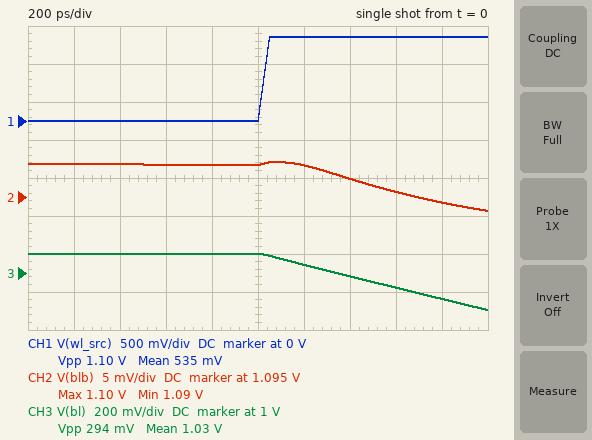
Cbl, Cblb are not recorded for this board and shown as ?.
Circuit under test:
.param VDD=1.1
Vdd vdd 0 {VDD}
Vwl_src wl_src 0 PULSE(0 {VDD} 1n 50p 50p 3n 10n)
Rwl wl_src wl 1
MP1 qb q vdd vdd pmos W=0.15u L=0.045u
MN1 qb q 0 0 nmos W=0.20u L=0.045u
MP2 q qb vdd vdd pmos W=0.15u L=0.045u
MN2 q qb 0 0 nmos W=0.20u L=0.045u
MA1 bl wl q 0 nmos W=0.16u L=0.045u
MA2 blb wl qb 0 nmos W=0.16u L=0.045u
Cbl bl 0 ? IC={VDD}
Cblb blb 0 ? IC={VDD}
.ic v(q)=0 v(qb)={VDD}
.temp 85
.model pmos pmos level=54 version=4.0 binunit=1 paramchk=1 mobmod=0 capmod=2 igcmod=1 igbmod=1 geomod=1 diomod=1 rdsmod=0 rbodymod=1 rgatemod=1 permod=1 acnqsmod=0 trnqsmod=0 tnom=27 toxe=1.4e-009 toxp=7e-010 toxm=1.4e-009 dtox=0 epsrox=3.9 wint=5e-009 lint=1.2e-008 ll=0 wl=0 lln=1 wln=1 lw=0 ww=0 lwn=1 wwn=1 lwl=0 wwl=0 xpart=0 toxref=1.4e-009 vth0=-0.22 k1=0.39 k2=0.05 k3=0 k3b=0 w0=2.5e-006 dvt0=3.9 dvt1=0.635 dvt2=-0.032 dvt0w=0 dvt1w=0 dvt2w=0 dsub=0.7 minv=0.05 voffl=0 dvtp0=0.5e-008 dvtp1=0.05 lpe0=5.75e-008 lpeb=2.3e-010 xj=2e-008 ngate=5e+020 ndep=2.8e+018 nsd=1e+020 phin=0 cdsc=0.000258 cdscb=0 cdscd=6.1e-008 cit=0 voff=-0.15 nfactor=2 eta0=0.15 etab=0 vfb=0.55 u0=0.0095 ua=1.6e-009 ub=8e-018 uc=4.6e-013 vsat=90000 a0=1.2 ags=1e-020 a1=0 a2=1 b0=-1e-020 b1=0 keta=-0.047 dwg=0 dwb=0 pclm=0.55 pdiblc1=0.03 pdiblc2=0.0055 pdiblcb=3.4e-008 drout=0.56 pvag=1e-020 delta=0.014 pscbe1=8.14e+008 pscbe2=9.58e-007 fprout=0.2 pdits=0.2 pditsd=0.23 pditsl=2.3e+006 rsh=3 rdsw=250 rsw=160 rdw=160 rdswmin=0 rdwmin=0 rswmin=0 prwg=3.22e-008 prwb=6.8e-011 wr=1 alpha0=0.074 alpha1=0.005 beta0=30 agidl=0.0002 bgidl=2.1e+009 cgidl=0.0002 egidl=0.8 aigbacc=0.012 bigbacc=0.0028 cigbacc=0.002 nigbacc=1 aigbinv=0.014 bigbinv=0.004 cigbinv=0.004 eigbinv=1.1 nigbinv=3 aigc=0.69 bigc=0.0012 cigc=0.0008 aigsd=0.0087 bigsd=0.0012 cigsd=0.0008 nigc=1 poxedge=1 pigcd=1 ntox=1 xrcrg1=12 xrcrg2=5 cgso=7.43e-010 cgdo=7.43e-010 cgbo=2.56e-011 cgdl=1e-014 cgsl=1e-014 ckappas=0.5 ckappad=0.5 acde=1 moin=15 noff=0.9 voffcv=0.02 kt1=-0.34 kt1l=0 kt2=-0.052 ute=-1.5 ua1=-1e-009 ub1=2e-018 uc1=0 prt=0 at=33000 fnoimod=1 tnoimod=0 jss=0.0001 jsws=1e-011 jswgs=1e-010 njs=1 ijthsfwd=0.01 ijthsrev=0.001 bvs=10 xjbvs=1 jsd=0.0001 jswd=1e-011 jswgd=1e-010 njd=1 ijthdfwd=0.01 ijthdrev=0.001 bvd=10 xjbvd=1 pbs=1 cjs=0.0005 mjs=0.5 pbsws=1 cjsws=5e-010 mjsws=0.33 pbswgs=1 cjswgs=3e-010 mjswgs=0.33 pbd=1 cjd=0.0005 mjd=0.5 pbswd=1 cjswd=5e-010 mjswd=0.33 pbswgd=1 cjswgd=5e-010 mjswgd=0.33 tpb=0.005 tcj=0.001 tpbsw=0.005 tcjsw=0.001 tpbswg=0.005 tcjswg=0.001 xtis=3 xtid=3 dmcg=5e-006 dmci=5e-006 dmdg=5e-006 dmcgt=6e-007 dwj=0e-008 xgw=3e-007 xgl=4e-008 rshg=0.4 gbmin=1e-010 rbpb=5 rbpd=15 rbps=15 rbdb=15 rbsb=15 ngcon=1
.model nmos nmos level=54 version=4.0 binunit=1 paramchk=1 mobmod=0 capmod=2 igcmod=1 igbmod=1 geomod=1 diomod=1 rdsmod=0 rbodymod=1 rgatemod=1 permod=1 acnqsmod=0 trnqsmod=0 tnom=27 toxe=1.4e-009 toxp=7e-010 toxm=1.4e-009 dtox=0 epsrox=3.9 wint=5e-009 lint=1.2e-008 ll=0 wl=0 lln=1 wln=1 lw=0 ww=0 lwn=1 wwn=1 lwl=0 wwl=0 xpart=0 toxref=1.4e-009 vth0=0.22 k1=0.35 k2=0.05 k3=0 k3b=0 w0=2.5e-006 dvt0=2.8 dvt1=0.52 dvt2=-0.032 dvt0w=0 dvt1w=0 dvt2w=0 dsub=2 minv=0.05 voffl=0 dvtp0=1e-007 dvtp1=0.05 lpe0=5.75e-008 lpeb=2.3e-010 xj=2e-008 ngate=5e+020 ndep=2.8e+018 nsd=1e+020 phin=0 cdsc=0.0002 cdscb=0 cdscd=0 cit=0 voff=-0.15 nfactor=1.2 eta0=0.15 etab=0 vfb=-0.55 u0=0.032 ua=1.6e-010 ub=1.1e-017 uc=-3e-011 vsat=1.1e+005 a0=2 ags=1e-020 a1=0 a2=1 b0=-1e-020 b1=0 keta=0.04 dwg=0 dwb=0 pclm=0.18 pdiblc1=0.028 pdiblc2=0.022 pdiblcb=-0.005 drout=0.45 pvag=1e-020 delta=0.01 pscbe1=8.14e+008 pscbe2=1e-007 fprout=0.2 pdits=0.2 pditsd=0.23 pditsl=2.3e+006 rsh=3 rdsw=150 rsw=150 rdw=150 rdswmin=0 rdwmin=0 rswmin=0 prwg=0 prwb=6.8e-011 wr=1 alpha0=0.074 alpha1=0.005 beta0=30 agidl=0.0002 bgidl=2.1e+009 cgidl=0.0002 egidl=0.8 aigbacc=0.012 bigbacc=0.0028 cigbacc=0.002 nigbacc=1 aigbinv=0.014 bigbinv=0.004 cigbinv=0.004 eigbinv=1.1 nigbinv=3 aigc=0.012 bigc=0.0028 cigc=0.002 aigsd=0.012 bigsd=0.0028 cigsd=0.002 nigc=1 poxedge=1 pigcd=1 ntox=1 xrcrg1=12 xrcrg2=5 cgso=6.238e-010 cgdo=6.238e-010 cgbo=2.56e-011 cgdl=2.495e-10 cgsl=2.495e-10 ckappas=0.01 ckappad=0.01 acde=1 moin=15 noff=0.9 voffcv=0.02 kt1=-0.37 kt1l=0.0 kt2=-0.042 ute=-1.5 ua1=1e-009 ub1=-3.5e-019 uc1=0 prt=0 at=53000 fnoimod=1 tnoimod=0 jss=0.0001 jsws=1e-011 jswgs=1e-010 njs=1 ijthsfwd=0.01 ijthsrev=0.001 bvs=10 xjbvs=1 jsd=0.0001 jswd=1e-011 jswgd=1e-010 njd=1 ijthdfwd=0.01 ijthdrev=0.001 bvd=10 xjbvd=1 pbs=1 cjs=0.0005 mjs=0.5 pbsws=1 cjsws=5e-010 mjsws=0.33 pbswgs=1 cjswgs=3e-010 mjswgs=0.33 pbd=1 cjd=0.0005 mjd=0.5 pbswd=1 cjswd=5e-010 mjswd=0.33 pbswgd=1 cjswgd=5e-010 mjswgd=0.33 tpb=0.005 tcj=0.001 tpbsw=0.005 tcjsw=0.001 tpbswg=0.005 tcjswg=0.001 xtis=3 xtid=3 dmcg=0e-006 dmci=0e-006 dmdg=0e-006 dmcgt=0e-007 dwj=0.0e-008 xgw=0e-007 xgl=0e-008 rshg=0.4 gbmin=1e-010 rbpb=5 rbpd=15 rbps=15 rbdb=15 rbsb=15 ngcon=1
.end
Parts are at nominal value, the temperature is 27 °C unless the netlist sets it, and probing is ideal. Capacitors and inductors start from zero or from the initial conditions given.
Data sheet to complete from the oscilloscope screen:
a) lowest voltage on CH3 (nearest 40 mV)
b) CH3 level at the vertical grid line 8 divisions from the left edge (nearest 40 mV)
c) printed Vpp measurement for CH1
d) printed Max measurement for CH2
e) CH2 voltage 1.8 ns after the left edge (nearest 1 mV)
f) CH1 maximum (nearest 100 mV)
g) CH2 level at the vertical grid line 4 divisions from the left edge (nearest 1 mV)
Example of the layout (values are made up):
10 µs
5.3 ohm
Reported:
800 mV
920 mV
1.10 V
1.10 V
1.094 V
1.1 V
1.099 V
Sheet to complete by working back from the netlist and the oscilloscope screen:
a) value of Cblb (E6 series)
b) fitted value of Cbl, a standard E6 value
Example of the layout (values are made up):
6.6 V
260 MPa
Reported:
330 fF
330 fF
